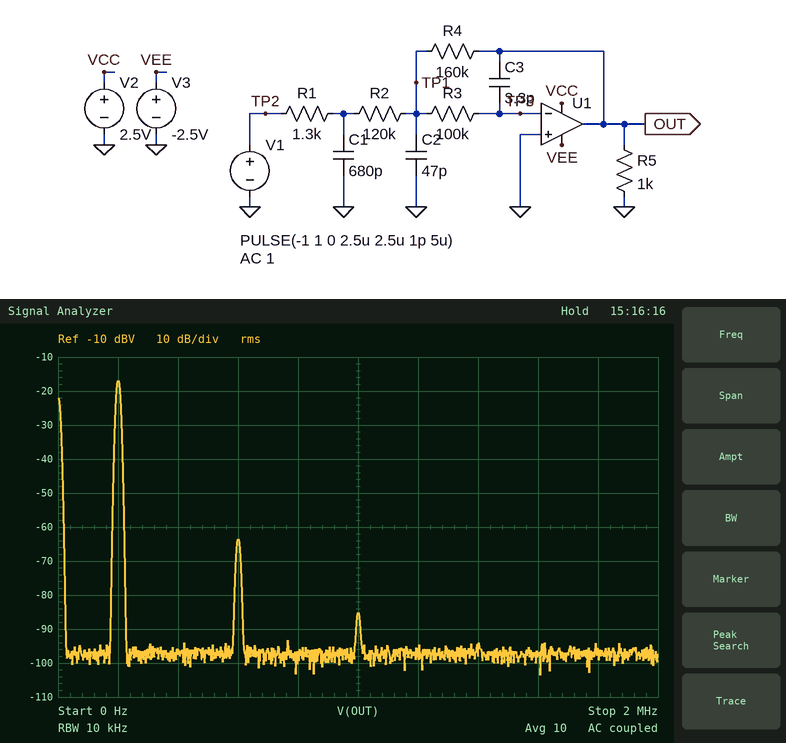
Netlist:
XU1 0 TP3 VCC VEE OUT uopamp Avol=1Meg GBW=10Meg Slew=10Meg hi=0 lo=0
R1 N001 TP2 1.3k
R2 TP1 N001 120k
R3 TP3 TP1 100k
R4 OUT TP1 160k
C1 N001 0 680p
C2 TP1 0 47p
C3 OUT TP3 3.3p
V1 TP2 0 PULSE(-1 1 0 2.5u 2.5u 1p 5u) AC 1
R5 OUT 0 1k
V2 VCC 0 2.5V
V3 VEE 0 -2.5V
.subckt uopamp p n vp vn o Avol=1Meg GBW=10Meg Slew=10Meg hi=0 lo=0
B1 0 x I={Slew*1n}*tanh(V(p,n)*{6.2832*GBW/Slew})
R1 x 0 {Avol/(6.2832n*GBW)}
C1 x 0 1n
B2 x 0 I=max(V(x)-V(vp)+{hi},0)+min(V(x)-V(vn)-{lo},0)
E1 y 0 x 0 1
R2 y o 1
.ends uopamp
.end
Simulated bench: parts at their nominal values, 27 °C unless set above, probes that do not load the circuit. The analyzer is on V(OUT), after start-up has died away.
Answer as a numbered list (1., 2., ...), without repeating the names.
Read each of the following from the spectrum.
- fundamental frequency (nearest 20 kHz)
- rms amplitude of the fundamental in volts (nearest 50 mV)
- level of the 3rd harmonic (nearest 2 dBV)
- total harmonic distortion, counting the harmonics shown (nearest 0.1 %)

1. 200 kHz
2. 150 mV
3. -64 dBV
4. 0.5 %
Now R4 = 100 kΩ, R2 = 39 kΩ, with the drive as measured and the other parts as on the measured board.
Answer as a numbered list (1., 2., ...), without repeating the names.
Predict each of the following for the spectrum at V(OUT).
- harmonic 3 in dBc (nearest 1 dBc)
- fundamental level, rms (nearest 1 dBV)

1. -46 dBc
2. -8 dBV
